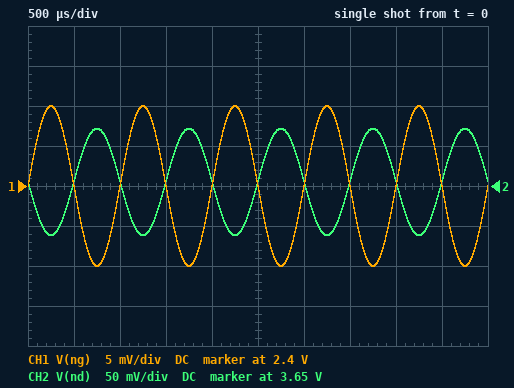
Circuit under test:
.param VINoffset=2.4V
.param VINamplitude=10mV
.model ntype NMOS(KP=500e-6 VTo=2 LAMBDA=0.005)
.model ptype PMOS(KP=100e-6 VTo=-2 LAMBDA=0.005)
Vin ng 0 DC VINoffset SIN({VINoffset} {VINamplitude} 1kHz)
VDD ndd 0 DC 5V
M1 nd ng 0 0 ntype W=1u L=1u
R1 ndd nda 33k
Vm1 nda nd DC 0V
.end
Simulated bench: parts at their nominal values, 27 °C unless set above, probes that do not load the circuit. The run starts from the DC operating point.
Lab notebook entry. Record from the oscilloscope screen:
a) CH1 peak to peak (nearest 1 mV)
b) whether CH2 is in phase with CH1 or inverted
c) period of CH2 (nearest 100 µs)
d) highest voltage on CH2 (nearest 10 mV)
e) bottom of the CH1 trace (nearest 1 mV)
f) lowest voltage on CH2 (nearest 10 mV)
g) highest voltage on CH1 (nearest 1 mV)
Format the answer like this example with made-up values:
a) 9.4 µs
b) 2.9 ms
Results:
a) 20 mV
b) inverted
c) 1.0 ms
d) 3.72 V
e) 2.390 V
f) 3.59 V
g) 2.410 V
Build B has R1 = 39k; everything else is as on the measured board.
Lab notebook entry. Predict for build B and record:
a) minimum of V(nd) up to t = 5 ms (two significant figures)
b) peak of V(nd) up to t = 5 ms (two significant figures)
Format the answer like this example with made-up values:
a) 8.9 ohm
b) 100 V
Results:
a) 3.3 V
b) 3.5 V
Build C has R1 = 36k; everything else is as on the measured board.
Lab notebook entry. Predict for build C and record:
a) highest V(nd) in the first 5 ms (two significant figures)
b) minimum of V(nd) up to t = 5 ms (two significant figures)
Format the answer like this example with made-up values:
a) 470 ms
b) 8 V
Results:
a) 3.6 V
b) 3.5 V
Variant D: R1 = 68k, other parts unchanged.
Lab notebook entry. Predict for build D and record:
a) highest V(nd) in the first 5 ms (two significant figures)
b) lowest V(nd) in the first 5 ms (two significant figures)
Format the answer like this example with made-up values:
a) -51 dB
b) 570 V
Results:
a) 2.4 V
b) 2.1 V
